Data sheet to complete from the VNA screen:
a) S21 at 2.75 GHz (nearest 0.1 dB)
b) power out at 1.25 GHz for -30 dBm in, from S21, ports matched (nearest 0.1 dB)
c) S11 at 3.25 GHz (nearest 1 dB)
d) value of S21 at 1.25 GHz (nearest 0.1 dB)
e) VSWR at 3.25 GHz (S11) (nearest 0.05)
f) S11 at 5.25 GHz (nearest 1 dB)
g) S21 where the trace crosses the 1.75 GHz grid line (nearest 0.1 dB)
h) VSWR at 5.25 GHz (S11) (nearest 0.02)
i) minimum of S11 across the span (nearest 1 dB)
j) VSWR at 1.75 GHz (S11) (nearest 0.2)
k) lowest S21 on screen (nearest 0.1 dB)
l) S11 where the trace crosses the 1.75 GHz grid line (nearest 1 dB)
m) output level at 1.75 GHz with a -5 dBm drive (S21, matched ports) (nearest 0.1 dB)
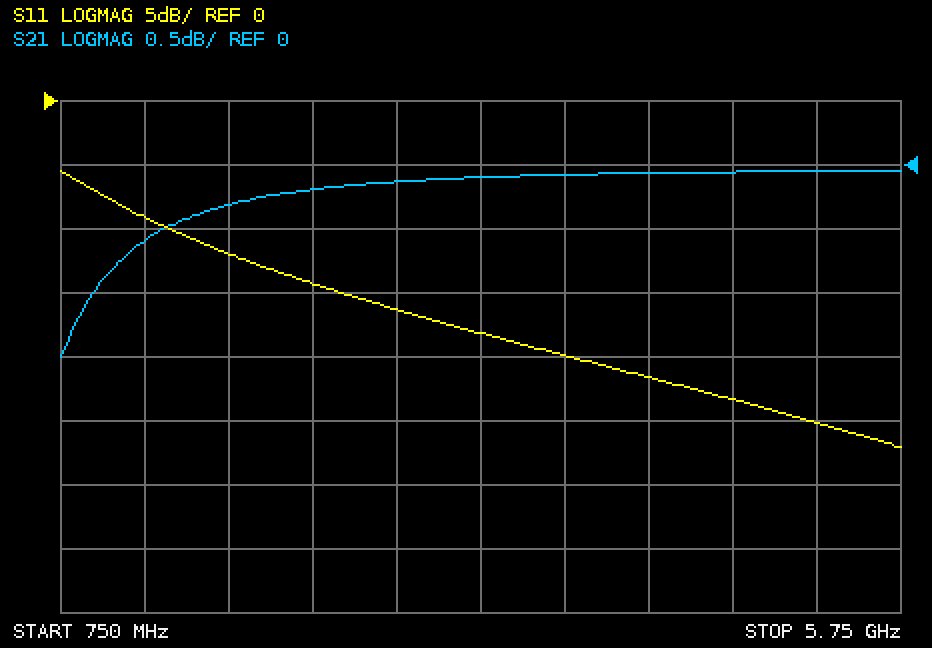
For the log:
-0.1 dB
-30.6 dBm
-18 dB
-0.6 dB
1.30
-25 dB
-0.3 dB
1.12
-27 dB
1.6
-1.5 dB
-12 dB
-5.3 dBm
